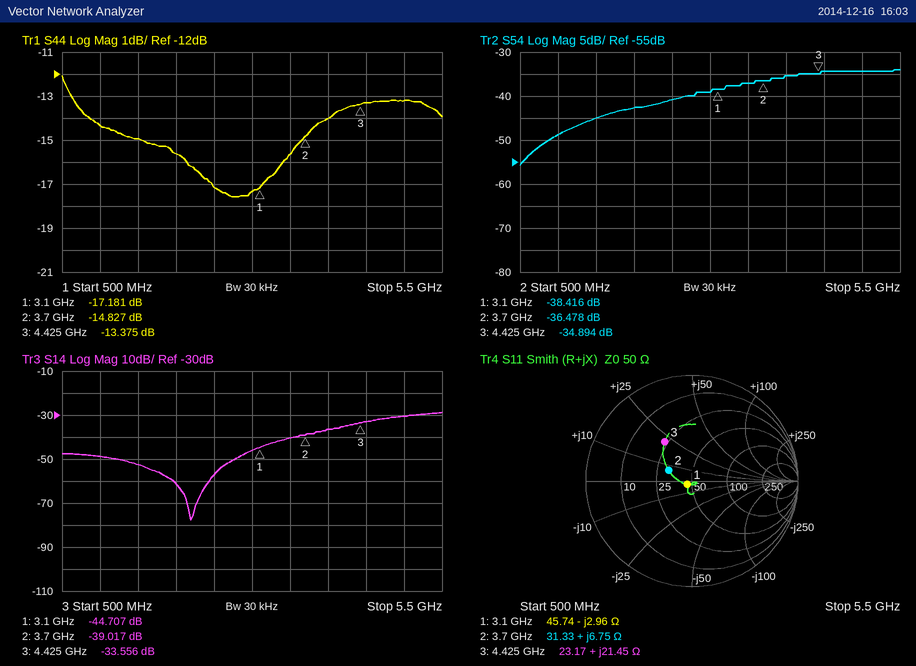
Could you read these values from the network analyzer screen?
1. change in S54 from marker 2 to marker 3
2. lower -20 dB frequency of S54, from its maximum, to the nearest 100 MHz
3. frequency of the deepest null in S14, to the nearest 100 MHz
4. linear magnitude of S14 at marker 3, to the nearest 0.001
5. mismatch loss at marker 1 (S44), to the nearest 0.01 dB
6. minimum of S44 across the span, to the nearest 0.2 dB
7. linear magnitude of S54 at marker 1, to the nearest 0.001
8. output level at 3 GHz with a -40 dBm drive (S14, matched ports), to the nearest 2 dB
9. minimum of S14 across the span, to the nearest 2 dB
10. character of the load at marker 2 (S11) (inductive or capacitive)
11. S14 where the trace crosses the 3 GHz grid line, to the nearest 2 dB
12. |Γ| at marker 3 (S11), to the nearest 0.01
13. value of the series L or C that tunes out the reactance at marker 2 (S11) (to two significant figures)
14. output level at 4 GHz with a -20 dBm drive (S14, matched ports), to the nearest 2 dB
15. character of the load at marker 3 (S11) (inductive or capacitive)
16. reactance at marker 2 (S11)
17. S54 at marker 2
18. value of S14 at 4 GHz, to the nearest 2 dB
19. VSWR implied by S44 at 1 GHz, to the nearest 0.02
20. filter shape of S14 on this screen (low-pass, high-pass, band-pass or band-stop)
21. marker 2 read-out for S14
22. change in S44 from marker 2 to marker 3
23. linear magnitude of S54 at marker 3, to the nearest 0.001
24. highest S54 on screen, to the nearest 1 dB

1.584 dB
600 MHz
2.2 GHz
0.021
0.08 dB
-17.6 dB
0.012
-86 dBm
-78 dB
inductive
-46 dB
0.45
6.4 pF
-56 dBm
inductive
+6.75 Ω
-36.478 dB
-36 dB
1.48
high-pass
-39.017 dB
1.452 dB
0.018
-34 dB
